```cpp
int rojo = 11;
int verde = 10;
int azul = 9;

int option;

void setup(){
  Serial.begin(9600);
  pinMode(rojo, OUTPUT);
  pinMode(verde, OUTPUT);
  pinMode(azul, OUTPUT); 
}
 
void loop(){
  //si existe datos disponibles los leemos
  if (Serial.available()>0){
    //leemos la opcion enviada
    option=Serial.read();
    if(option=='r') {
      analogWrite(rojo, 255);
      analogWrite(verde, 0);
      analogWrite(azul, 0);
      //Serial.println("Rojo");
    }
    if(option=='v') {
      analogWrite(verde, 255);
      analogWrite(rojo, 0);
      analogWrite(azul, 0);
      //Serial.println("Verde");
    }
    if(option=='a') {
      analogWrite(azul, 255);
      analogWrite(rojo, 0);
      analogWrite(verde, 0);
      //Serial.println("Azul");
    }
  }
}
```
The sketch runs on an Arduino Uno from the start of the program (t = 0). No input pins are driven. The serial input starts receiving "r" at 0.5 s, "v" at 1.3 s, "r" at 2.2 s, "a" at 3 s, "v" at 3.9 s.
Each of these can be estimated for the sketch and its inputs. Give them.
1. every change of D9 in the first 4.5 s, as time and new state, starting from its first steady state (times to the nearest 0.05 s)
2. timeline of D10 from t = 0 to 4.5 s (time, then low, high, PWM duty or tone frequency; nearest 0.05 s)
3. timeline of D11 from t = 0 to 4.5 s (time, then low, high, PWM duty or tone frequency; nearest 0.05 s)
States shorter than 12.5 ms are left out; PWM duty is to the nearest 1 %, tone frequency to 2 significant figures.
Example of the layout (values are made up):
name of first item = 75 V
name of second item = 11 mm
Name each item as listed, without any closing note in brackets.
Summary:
every change of D9 in the first 4.5 s, as time and new state, starting from its first steady state = 0 s low; 3 s high; 3.9 s low
timeline of D10 from t = 0 to 4.5 s = 0 s low; 1.3 s high; 2.2 s low; 3.9 s high
timeline of D11 from t = 0 to 4.5 s = 0 s low; 0.5 s high; 1.3 s low; 2.2 s high; 3 s low
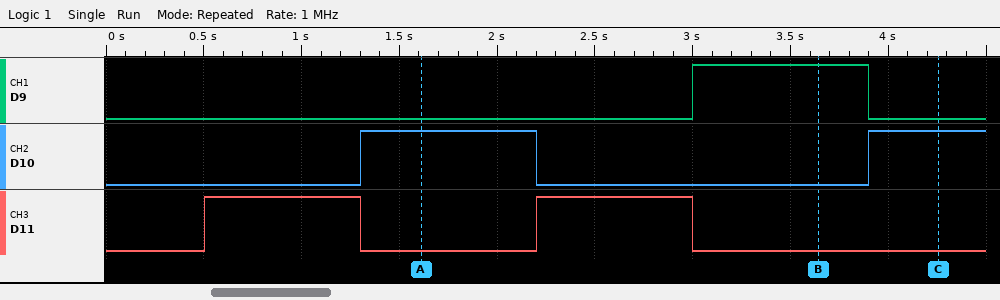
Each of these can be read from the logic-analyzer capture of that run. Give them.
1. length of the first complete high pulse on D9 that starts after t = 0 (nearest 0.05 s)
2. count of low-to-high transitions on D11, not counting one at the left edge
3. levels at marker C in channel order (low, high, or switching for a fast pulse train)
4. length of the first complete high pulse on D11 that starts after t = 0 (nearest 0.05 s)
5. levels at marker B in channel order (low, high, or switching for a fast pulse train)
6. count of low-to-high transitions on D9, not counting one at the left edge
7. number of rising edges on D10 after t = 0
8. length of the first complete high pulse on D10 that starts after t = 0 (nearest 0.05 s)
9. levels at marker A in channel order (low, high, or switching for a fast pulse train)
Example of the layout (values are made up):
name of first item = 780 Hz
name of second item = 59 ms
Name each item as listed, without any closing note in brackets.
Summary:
length of the first complete high pulse on D9 that starts after t = 0 = 0.90 s
count of low-to-high transitions on D11, not counting one at the left edge = 2
levels at marker C in channel order = D9 low, D10 high, D11 low
length of the first complete high pulse on D11 that starts after t = 0 = 0.80 s
levels at marker B in channel order = D9 high, D10 low, D11 low
count of low-to-high transitions on D9, not counting one at the left edge = 1
number of rising edges on D10 after t = 0 = 2
length of the first complete high pulse on D10 that starts after t = 0 = 0.90 s
levels at marker A in channel order = D9 low, D10 high, D11 low
